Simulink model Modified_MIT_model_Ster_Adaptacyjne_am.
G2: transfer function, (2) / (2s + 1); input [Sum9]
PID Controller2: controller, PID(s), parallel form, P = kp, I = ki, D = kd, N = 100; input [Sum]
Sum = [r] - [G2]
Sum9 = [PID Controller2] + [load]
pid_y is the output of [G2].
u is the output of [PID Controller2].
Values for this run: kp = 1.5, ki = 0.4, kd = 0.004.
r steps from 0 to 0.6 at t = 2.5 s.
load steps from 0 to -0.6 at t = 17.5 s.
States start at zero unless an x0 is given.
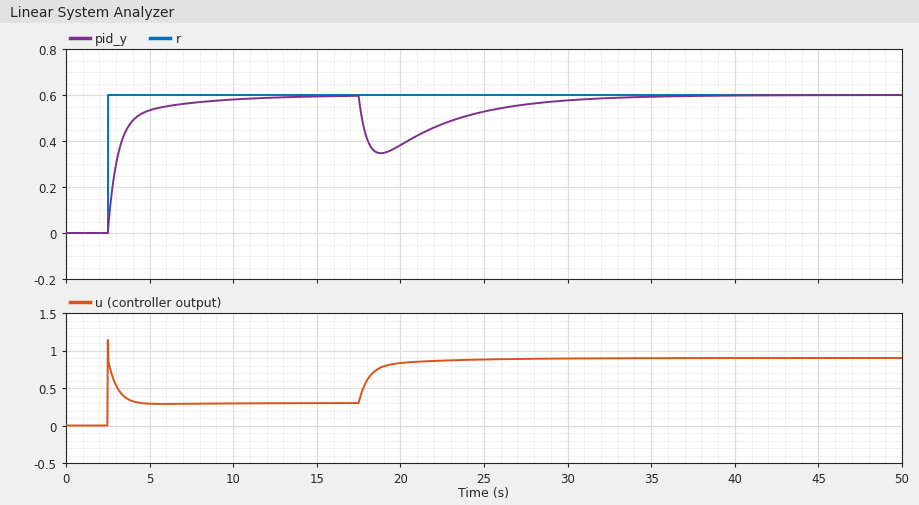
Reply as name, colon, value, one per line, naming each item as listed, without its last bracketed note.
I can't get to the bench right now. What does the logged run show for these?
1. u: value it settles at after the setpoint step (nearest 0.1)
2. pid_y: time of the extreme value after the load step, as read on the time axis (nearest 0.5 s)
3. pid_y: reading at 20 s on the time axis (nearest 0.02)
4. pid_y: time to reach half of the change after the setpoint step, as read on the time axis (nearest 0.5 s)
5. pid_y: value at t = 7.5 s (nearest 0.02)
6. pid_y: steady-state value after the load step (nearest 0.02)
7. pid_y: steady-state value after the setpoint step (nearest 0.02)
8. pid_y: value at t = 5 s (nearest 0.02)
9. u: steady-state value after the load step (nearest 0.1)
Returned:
u: value it settles at after the setpoint step: 0.3
pid_y: time of the extreme value after the load step, as read on the time axis: 19.0 s
pid_y: reading at 20 s on the time axis: 0.38
pid_y: time to reach half of the change after the setpoint step, as read on the time axis: 3.0 s
pid_y: value at t = 7.5 s: 0.56
pid_y: steady-state value after the load step: 0.60
pid_y: steady-state value after the setpoint step: 0.60
pid_y: value at t = 5 s: 0.54
u: steady-state value after the load step: 0.9
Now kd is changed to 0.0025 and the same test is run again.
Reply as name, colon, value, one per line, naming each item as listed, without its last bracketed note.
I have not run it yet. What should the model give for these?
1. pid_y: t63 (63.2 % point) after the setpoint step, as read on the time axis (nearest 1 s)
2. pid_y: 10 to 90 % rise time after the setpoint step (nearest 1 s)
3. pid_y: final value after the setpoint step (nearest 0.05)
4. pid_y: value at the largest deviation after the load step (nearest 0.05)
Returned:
pid_y: t63 (63.2 % point) after the setpoint step, as read on the time axis: 3 s
pid_y: 10 to 90 % rise time after the setpoint step: 3 s
pid_y: final value after the setpoint step: 0.60
pid_y: value at the largest deviation after the load step: 0.35
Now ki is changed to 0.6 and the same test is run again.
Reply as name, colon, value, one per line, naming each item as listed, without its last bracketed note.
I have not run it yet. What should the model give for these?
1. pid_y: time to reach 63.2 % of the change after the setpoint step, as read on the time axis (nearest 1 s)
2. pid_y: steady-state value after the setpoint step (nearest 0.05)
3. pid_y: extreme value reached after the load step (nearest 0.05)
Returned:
pid_y: time to reach 63.2 % of the change after the setpoint step, as read on the time axis: 3 s
pid_y: steady-state value after the setpoint step: 0.60
pid_y: extreme value reached after the load step: 0.35
